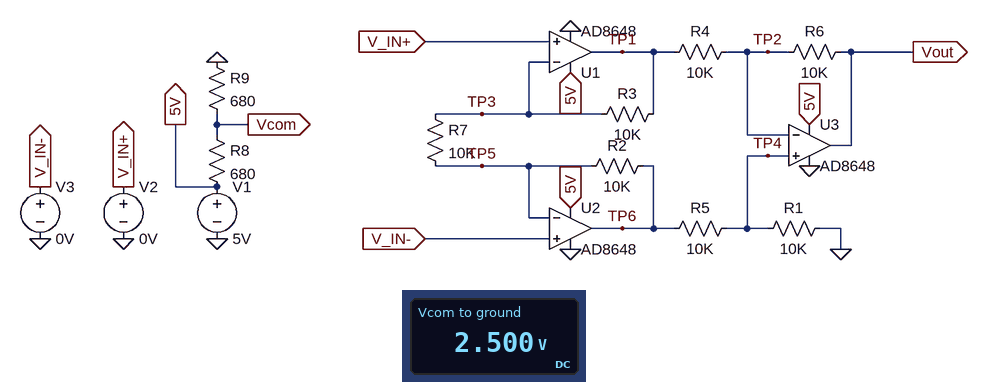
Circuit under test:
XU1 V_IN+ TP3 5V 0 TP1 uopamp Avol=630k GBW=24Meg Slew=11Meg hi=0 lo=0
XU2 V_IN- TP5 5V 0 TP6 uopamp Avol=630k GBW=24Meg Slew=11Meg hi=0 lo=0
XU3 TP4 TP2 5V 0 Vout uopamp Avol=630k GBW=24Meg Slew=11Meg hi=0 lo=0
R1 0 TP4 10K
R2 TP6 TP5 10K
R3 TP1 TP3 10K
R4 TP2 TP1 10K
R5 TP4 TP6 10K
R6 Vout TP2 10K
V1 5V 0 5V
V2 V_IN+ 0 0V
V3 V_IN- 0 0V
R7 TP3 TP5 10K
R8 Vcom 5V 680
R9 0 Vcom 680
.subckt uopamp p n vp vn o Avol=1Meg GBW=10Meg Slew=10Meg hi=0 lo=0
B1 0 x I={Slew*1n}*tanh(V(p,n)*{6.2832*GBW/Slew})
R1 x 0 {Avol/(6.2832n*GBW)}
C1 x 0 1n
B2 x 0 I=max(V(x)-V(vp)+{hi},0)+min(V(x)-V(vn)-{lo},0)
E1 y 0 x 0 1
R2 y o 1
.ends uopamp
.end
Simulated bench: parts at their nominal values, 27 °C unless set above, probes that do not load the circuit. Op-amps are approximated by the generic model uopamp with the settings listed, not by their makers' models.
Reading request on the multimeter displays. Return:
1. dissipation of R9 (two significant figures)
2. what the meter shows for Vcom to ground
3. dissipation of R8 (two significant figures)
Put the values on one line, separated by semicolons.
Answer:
9.2 mW; 2.500 V; 9.2 mW
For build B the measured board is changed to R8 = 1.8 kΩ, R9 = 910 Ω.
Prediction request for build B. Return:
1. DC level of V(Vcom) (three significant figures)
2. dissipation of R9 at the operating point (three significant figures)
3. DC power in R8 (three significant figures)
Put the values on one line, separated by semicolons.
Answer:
1.68 V; 3.10 mW; 6.13 mW
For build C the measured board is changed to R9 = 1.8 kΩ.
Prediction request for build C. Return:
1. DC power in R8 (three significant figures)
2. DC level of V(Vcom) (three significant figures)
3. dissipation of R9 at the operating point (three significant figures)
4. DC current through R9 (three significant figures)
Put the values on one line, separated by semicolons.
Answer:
2.76 mW; 3.63 V; 7.32 mW; 2.02 mA
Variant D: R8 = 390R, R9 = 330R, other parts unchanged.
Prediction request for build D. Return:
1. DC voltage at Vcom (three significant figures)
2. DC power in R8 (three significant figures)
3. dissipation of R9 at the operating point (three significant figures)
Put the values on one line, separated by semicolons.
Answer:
2.29 V; 18.8 mW; 15.9 mW
